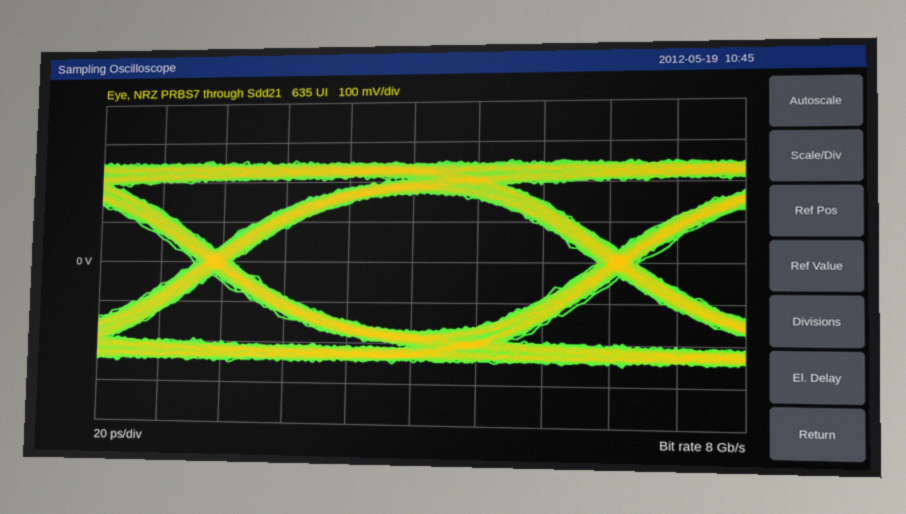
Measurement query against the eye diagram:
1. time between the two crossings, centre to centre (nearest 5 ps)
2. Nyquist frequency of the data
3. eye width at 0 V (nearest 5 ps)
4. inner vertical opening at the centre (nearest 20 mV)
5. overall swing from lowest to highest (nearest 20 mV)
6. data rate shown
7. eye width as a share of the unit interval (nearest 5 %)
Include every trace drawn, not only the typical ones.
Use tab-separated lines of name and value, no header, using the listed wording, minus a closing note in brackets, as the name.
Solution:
time between the two crossings, centre to centre	125 ps
Nyquist frequency of the data	4 GHz
eye width at 0 V	115 ps
inner vertical opening at the centre	340 mV
overall swing from lowest to highest	500 mV
data rate shown	8 Gb/s
eye width as a share of the unit interval	90 %
